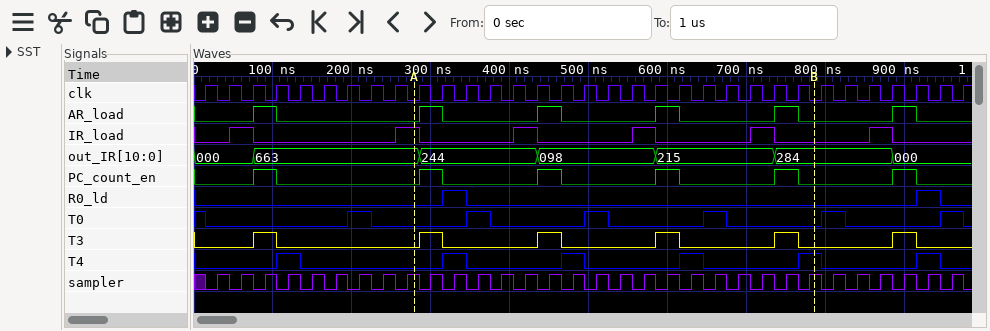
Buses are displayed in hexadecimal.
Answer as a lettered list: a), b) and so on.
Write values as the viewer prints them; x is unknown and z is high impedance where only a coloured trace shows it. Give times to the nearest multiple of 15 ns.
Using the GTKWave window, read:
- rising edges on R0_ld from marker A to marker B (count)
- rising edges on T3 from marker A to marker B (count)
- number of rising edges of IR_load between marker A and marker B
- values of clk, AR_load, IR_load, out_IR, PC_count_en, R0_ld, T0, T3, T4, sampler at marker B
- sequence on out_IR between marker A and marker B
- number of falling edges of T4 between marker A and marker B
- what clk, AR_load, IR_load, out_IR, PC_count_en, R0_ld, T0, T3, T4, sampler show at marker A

a) 1
b) 4
c) 3
d) clk=0, AR_load=0, IR_load=0, out_IR=284, PC_count_en=0, R0_ld=0, T0=0, T3=0, T4=1, sampler=1
e) 663, 244, 098, 215, 284
f) 3
g) clk=0, AR_load=0, IR_load=1, out_IR=663, PC_count_en=0, R0_ld=0, T0=0, T3=0, T4=0, sampler=1
